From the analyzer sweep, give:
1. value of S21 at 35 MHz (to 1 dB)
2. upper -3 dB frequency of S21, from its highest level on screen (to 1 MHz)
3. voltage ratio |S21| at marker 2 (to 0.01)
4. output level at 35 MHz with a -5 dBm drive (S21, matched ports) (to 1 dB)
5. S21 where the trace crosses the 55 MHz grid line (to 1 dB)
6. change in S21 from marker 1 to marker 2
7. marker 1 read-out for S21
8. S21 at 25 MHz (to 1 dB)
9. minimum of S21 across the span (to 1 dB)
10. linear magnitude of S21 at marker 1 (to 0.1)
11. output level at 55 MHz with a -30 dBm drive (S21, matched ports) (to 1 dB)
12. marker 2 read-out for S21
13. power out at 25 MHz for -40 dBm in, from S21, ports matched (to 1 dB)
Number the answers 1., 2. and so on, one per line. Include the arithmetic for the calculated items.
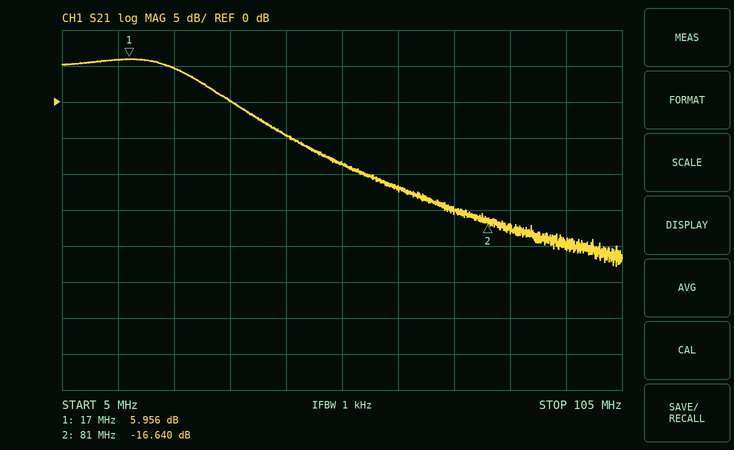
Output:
1. 0 dB
2. 29 MHz
3. 10^(-16.64/20) ≈ 0.15
4. -5 dBm + (0 dB) = -5 dBm
5. -9 dB
6. -16.64 − (5.956) = -22.596 dB
7. 5.956 dB
8. 5 dB
9. -23 dB
10. 10^(5.956/20) ≈ 2.0
11. -30 dBm + (-9 dB) = -39 dBm
12. -16.640 dB
13. -40 dBm + (5 dB) = -35 dBm
